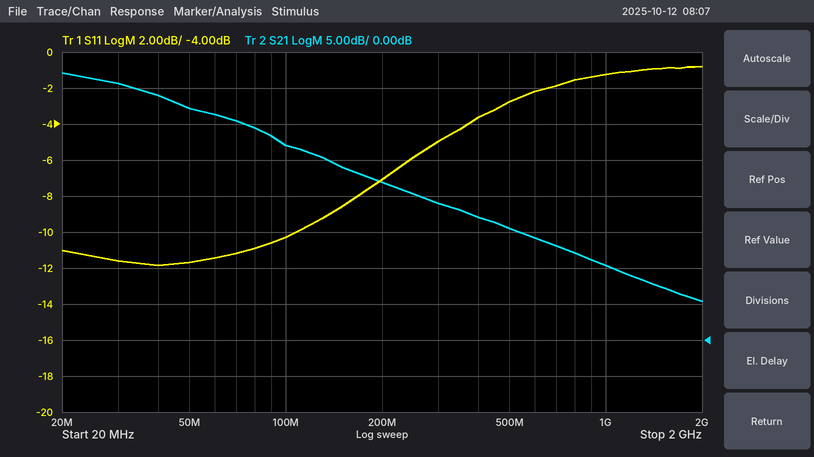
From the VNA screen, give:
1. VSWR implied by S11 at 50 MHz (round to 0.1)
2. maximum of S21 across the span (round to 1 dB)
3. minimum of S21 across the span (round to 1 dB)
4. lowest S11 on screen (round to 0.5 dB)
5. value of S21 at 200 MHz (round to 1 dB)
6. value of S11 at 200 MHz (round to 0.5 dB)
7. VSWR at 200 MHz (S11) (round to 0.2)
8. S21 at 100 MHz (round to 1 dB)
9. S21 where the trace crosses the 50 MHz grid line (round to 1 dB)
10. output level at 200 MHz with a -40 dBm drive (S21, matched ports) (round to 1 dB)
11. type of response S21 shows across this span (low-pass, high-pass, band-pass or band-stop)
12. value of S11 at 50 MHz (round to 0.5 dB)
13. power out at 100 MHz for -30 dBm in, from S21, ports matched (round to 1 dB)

1.7
37 dB
5 dB
-12.0 dB
22 dB
-7.0 dB
2.6
27 dB
32 dB
-18 dBm
low-pass
-11.5 dB
-3 dBm
